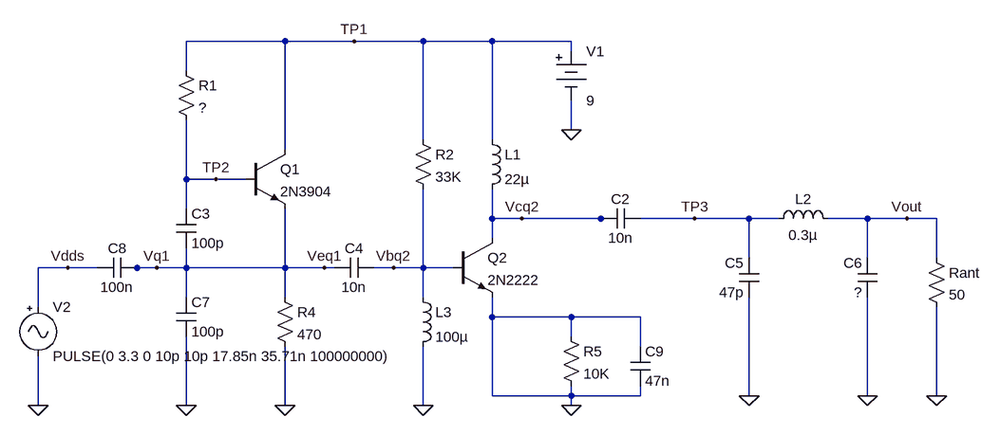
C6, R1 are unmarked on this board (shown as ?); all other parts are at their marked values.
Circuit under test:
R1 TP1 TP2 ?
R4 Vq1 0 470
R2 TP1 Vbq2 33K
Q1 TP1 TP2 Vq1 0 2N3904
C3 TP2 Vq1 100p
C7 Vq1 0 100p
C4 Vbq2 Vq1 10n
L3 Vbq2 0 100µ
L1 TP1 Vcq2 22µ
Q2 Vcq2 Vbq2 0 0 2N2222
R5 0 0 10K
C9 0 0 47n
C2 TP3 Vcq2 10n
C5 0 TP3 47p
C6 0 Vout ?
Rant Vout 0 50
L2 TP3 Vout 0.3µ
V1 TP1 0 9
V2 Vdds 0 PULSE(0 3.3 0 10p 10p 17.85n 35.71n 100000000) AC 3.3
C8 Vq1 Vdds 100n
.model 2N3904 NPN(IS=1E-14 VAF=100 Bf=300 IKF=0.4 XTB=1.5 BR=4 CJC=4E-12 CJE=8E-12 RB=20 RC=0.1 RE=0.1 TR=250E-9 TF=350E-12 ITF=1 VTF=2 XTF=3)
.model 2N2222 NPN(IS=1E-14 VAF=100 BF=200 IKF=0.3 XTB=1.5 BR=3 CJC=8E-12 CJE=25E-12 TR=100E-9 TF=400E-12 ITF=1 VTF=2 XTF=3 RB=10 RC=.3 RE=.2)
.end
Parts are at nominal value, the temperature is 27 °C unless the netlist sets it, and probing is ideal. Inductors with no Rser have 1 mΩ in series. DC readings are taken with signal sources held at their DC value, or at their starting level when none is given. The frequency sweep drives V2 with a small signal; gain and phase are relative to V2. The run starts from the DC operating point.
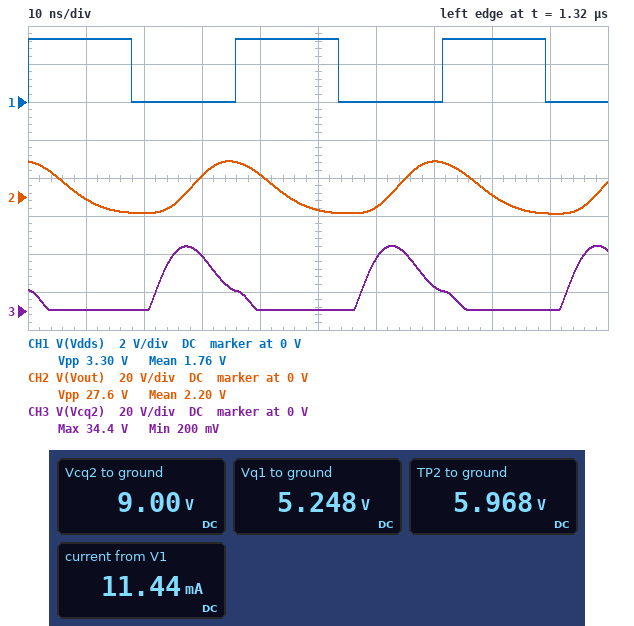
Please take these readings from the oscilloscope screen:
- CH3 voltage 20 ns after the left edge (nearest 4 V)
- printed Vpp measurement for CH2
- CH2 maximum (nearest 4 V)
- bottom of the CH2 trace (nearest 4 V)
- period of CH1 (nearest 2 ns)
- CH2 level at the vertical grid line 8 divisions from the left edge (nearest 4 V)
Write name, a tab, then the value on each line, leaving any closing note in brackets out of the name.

CH3 voltage 20 ns after the left edge	0 V
printed Vpp measurement for CH2	27.6 V
CH2 maximum	20 V
bottom of the CH2 trace	-8 V
period of CH1	36 ns
CH2 level at the vertical grid line 8 divisions from the left edge	0 V
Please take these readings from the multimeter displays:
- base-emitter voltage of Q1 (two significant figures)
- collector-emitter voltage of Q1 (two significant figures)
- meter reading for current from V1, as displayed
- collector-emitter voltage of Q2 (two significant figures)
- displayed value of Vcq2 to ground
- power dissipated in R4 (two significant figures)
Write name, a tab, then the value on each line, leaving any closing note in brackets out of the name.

base-emitter voltage of Q1	720 mV
collector-emitter voltage of Q1	3.8 V
meter reading for current from V1, as displayed	11.44 mA
collector-emitter voltage of Q2	9.0 V
displayed value of Vcq2 to ground	9.00 V
power dissipated in R4	59 mW
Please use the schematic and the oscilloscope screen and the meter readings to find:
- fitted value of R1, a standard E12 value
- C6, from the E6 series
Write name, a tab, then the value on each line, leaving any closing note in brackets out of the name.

fitted value of R1, a standard E12 value	82 kΩ
C6, from the E6 series	68 pF
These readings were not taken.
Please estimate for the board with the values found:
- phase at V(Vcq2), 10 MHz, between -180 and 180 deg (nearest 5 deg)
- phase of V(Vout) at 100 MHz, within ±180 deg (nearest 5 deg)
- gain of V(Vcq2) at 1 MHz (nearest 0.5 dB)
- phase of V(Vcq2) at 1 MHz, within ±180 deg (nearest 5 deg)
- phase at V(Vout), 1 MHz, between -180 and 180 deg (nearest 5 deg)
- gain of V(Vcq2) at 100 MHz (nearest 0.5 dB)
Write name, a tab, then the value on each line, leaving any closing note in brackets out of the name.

phase at V(Vcq2), 10 MHz, between -180 and 180 deg	90 deg
phase of V(Vout) at 100 MHz, within ±180 deg	-160 deg
gain of V(Vcq2) at 1 MHz	-58.5 dB
phase of V(Vcq2) at 1 MHz, within ±180 deg	95 deg
phase at V(Vout), 1 MHz, between -180 and 180 deg	110 deg
gain of V(Vcq2) at 100 MHz	-21.5 dB
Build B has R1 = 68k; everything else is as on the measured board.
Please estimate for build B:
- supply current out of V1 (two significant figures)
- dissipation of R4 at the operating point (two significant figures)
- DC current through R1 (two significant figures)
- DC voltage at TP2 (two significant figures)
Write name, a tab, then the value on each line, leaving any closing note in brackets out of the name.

supply current out of V1	12 mA
dissipation of R4 at the operating point	66 mW
DC current through R1	40 µA
DC voltage at TP2	6.3 V
